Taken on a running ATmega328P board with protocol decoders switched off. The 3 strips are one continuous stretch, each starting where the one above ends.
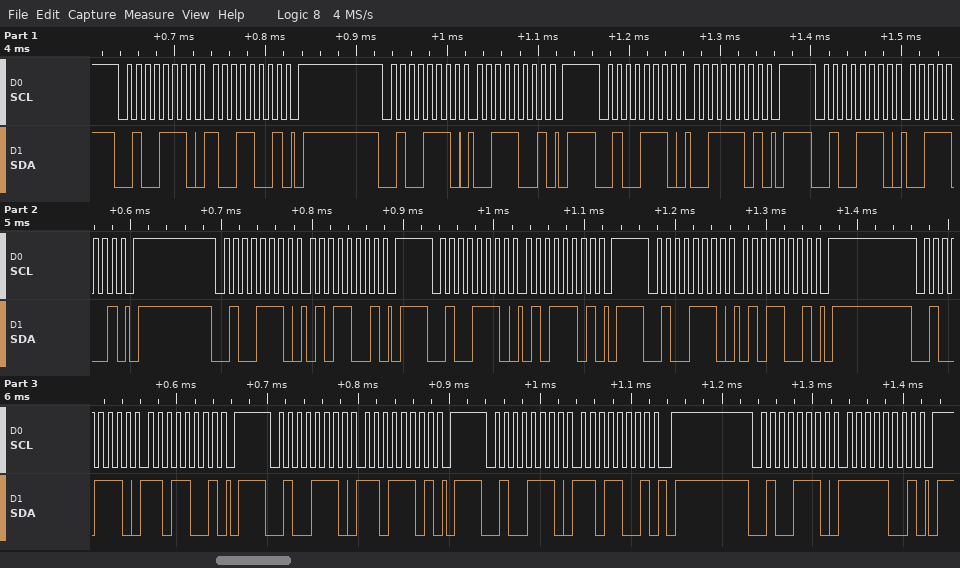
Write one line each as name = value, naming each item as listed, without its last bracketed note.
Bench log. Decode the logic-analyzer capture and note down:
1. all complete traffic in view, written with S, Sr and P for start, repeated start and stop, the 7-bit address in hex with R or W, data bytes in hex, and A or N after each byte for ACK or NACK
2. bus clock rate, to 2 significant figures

all complete traffic in view, written with S, Sr and P for start, repeated start and stop, the 7-bit address in hex with R or W, data bytes in hex, and A or N after each byte for ACK or NACK = S 27W A 99 A P S 27W A 39 A P S 27W A 3D A P S 27W A 39 A P S 27W A 59 A P S 27W A 5D A P S 27W A 59 A P S 27W A D9 A P S 27W A DD A P S 27W A D9 A P S 27W A F9 A P
bus clock rate, to 2 significant figures = 100 kHz
